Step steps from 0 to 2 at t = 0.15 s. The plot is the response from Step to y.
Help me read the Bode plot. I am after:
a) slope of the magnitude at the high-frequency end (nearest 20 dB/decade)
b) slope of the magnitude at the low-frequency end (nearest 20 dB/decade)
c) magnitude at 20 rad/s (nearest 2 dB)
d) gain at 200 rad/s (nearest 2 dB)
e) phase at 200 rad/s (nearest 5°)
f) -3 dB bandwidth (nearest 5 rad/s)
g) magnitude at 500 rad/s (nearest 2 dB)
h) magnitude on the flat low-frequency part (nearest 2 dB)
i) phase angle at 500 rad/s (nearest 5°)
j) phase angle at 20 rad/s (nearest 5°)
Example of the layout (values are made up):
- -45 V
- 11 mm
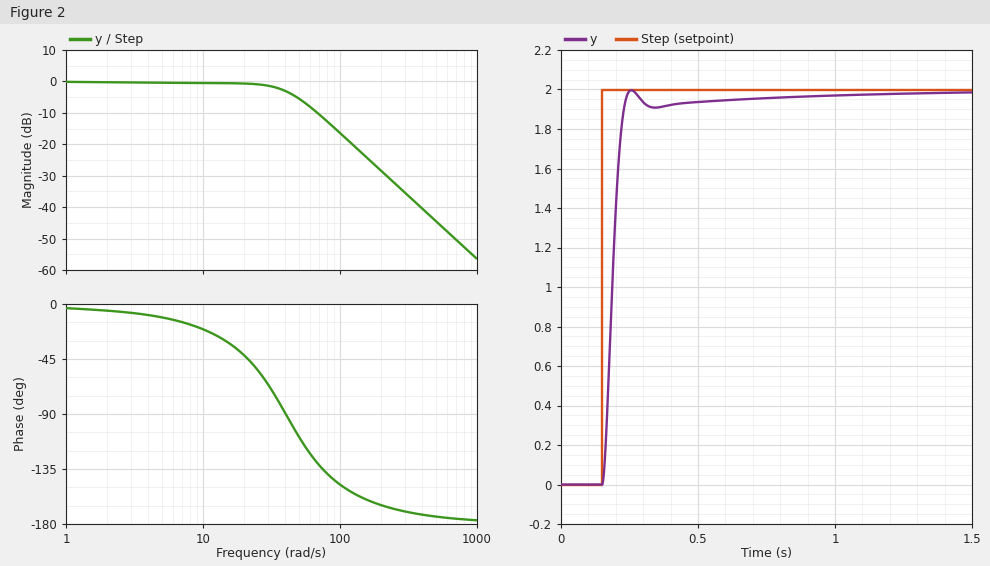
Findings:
- -40 dB/decade
- 0 dB/decade
- 0 dB
- -28 dB
- -165°
- 40 rad/s
- -44 dB
- 0 dB
- -175°
- -40°
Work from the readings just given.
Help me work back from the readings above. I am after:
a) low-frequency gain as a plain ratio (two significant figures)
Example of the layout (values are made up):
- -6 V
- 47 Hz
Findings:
- 1.0
